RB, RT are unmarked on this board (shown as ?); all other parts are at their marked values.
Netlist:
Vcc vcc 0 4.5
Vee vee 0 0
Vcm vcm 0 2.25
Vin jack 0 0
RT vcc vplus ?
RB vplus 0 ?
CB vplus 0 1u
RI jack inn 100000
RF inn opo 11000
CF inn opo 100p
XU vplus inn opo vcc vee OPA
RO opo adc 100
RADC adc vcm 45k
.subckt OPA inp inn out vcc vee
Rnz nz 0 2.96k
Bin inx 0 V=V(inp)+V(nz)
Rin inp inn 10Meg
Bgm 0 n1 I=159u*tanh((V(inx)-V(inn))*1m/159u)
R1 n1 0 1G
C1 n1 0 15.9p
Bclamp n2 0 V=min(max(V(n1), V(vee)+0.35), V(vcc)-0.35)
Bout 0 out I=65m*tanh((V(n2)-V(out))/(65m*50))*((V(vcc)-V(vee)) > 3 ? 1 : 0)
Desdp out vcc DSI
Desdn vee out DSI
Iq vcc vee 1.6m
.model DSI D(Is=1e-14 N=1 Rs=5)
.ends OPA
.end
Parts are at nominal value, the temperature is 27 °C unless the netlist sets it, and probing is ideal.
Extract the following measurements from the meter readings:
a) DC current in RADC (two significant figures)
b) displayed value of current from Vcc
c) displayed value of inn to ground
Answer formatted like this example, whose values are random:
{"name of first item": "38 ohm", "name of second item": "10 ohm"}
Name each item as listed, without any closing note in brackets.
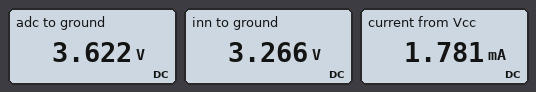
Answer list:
{"DC current in RADC": "30 µA", "displayed value of current from Vcc": "1.781 mA", "displayed value of inn to ground": "3.266 V"}
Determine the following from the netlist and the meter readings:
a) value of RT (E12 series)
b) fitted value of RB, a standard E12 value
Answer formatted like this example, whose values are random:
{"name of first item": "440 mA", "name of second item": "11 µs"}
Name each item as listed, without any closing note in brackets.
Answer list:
{"value of RT": "6.8 kΩ", "fitted value of RB, a standard E12 value": "18 kΩ"}
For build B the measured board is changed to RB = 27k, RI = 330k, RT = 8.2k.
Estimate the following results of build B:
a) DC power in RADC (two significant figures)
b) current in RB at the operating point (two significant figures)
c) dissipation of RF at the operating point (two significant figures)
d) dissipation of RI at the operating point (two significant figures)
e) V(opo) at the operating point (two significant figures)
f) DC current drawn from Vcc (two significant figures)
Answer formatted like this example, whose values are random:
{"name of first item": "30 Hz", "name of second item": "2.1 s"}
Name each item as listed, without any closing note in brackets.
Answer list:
{"DC power in RADC": "38 µW", "current in RB at the operating point": "130 µA", "dissipation of RF at the operating point": "1.2 µW", "dissipation of RI at the operating point": "36 µW", "V(opo) at the operating point": "3.6 V", "DC current drawn from Vcc": "1.7 mA"}
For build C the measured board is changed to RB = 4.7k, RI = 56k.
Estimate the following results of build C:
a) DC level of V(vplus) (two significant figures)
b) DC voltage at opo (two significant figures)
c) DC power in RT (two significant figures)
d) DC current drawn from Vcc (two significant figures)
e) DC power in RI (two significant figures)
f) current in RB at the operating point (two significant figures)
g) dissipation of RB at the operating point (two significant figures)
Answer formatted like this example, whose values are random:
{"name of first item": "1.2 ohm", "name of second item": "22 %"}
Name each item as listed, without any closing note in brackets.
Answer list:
{"DC level of V(vplus)": "1.8 V", "DC voltage at opo": "2.2 V", "DC power in RT": "1.0 mW", "DC current drawn from Vcc": "2.0 mA", "DC power in RI": "60 µW", "current in RB at the operating point": "390 µA", "dissipation of RB at the operating point": "720 µW"}
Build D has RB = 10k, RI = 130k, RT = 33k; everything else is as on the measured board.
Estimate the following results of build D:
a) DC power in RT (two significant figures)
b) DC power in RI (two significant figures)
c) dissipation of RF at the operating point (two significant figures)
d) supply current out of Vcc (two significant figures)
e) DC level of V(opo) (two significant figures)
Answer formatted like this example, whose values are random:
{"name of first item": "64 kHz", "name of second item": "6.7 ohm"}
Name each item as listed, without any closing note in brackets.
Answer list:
{"DC power in RT": "360 µW", "DC power in RI": "8.4 µW", "dissipation of RF at the operating point": "710 nW", "supply current out of Vcc": "1.7 mA", "DC level of V(opo)": "1.1 V"}
